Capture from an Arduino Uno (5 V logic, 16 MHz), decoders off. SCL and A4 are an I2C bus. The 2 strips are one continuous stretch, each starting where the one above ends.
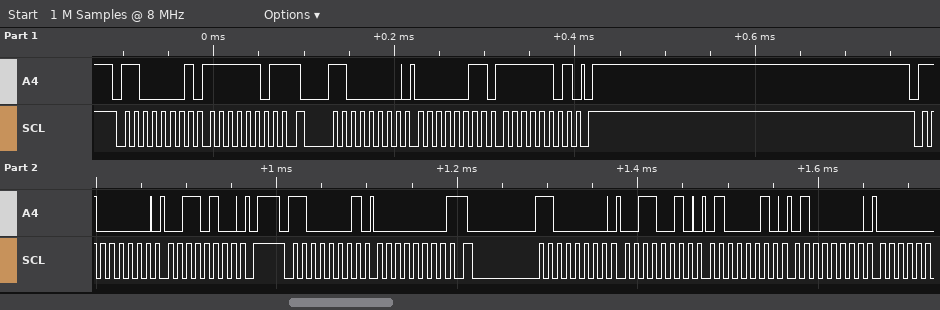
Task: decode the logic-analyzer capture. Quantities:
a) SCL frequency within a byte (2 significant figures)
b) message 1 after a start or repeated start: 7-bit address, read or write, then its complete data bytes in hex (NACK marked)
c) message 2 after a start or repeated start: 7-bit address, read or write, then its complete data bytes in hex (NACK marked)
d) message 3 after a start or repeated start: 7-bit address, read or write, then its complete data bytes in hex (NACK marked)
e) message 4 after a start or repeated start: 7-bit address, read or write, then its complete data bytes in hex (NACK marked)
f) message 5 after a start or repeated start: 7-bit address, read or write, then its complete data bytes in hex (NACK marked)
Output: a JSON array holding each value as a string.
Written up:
["100 kHz", "0x60 read: FD NACK", "0x60 write: 03 FD", "0x60 write: 34", "0x60 read: 00 NACK", "0x60 write: 32 42 40"]
